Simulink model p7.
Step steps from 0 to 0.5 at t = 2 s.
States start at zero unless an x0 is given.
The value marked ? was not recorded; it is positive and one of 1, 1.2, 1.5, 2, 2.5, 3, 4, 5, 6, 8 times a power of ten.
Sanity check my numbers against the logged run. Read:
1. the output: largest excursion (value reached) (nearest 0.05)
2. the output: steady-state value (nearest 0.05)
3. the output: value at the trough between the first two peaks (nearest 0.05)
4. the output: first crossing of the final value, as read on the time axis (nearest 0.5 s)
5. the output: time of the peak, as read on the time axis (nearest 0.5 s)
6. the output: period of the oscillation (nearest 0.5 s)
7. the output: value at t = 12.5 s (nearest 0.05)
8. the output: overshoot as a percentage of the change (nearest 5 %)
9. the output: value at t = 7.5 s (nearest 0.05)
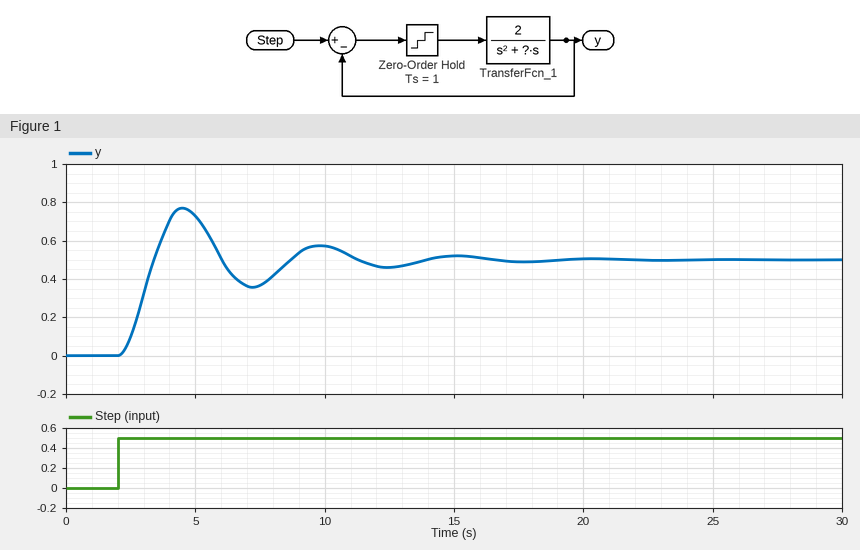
0.75
0.50
0.35
3.5 s
4.5 s
5.5 s
0.45
55 %
0.35
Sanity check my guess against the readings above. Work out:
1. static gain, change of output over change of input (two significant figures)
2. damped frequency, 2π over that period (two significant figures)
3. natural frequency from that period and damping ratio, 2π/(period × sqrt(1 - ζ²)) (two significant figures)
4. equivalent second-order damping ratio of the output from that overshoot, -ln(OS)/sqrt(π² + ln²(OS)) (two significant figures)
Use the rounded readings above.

1.0
1.1 rad/s
1.2 rad/s
0.19
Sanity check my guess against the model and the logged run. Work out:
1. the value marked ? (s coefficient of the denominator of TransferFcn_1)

1.5
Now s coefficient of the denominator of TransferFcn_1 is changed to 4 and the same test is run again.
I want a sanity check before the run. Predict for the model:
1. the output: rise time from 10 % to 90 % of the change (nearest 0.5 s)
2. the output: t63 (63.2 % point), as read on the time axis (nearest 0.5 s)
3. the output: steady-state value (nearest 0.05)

2.5 s
3.5 s
0.50
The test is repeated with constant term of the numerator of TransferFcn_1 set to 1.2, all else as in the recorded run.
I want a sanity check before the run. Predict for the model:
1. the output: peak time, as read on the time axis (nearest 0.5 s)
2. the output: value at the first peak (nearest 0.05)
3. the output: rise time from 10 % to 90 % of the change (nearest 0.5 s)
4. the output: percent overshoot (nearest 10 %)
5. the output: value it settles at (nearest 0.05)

5.5 s
0.65
1.5 s
30 %
0.50
